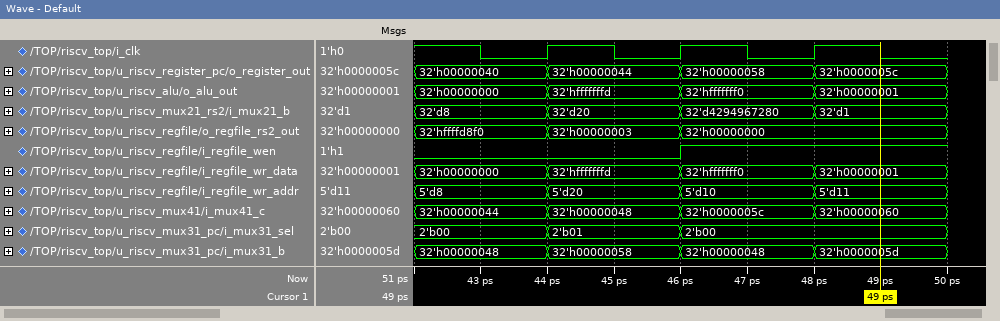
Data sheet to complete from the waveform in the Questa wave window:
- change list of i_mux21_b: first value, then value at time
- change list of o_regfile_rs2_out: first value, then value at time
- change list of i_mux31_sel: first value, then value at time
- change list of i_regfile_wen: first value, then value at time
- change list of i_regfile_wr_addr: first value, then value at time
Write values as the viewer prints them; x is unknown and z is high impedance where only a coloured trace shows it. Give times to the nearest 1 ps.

32'd8, 32'd20 at 44 ps, 32'd4294967280 at 46 ps, 32'd1 at 48 ps
32'hffffd8f0, 32'h00000003 at 44 ps, 32'h00000000 at 46 ps
2'b00, 2'b01 at 44 ps, 2'b00 at 46 ps
0, 1 at 46 ps
5'd8, 5'd20 at 44 ps, 5'd10 at 46 ps, 5'd11 at 48 ps
